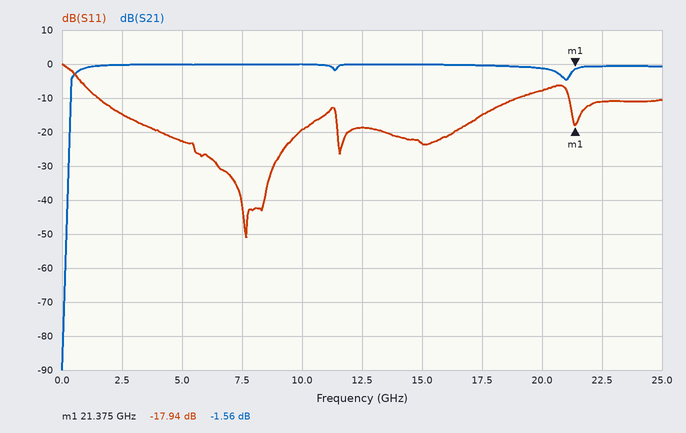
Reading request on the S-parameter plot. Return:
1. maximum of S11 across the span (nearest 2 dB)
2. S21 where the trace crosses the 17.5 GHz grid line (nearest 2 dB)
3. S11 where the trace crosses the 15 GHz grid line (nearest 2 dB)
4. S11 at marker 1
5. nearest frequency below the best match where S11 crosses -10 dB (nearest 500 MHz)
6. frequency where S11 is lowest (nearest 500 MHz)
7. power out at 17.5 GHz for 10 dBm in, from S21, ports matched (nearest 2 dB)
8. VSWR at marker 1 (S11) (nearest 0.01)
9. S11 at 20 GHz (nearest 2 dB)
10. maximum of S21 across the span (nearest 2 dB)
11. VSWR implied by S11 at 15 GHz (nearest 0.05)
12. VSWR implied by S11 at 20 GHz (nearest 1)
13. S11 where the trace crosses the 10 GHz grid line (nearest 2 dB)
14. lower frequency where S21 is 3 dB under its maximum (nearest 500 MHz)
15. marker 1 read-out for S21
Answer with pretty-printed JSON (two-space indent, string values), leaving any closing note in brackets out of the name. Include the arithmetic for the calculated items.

{
  "maximum of S11 across the span": "0 dB",
  "S21 where the trace crosses the 17.5 GHz grid line": "0 dB",
  "S11 where the trace crosses the 15 GHz grid line": "-24 dB",
  "S11 at marker 1": "-17.94 dB",
  "nearest frequency below the best match where S11 crosses -10 dB": "1.5 GHz",
  "frequency where S11 is lowest": "7.5 GHz",
  "power out at 17.5 GHz for 10 dBm in, from S21, ports matched": "10 dBm + (0 dB) = 10 dBm",
  "VSWR at marker 1 (S11)": "(1 + 0.1268)/(1 − 0.1268) ≈ 1.29",
  "S11 at 20 GHz": "-8 dB",
  "maximum of S21 across the span": "0 dB",
  "VSWR implied by S11 at 15 GHz": "|Γ| = 10^(-24/20) = 0.0631; VSWR = (1 + 0.0631)/(1 − 0.0631) ≈ 1.13, so 1.15 to the nearest 0.05",
  "VSWR implied by S11 at 20 GHz": "|Γ| = 10^(-8/20) = 0.3981; VSWR = (1 + 0.3981)/(1 − 0.3981) ≈ 2",
  "S11 where the trace crosses the 10 GHz grid line": "-20 dB",
  "lower frequency where S21 is 3 dB under its maximum": "500 MHz",
  "marker 1 read-out for S21": "-1.56 dB"
}
